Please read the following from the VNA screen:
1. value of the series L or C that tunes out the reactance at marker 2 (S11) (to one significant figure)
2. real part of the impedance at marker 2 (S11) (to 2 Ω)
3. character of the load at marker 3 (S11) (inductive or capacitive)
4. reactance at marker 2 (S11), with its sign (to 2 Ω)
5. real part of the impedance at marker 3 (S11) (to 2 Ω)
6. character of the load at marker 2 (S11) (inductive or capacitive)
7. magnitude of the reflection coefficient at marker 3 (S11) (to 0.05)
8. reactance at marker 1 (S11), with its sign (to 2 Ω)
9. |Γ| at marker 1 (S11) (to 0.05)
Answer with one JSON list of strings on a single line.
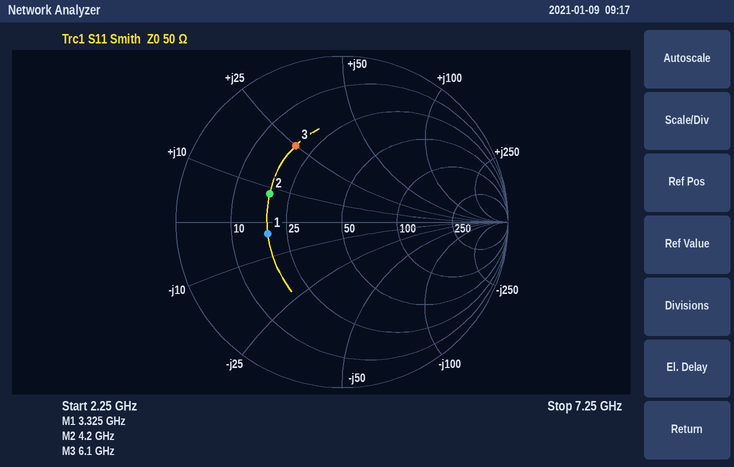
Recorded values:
["5 pF", "18 Ω", "inductive", "+8 Ω", "20 Ω", "inductive", "0.55", "-4 Ω", "0.45"]
